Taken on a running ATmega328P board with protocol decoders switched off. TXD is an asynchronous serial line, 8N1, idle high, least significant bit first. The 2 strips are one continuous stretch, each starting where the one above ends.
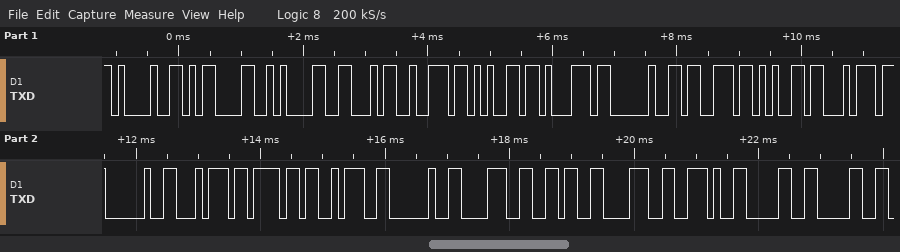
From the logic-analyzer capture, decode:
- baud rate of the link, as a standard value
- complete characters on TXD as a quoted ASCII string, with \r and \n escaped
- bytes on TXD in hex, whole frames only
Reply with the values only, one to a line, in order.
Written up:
9600 baud
"!\r\nFreq set to: 868.00"
21 0D 0A 46 72 65 71 20 73 65 74 20 74 6F 3A 20 38 36 38 2E 30 30
